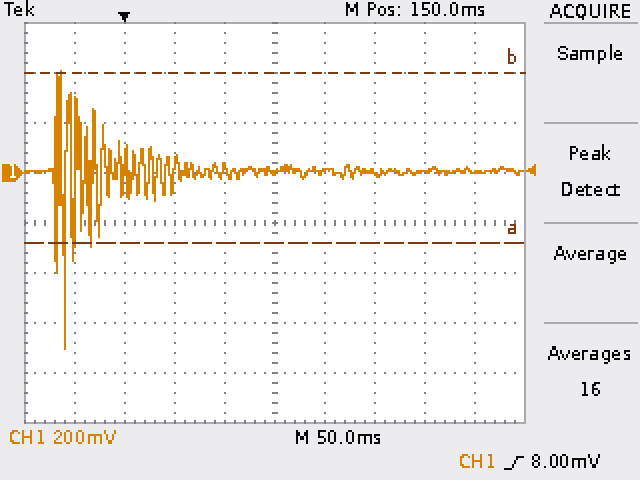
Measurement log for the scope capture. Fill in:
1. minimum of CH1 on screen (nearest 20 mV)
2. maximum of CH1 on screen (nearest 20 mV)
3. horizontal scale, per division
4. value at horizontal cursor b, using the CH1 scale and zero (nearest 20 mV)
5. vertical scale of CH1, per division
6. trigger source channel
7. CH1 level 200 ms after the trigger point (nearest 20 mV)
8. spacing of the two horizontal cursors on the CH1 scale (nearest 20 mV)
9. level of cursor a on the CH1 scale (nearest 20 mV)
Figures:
-700 mV
400 mV
50 ms
400 mV
200 mV
CH1
0 mV
680 mV
-280 mV
